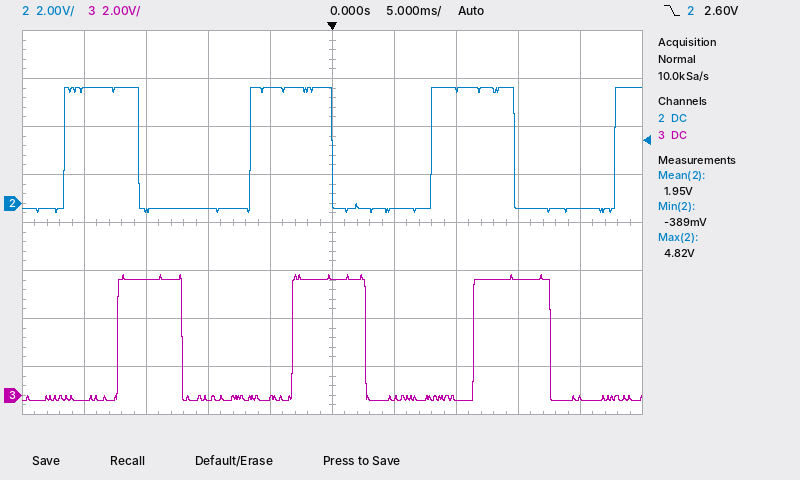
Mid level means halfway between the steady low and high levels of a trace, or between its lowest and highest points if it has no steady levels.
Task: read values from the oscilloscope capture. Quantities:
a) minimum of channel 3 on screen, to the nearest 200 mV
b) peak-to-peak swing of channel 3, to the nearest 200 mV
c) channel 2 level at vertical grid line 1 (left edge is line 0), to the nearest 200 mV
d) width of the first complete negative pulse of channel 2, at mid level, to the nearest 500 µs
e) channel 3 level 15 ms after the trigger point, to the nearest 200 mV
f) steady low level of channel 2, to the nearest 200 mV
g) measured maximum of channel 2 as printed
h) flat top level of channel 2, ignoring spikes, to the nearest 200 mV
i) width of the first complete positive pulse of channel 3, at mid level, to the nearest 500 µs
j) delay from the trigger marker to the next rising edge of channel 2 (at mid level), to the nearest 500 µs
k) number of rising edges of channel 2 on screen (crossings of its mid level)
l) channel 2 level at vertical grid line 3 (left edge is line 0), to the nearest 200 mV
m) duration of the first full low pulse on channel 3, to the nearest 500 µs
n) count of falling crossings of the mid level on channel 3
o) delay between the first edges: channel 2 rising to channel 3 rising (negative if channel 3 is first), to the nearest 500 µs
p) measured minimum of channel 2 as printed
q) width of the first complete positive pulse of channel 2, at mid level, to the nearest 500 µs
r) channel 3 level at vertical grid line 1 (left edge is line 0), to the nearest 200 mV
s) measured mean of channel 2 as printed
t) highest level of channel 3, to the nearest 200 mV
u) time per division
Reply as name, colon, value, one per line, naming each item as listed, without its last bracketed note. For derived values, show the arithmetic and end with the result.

minimum of channel 3 on screen, to the nearest 200 mV: -200 mV
peak-to-peak swing of channel 3, to the nearest 200 mV: 5.0 V − (-200 mV) = 5.2 V
channel 2 level at vertical grid line 1 (left edge is line 0), to the nearest 200 mV: 4.8 V
width of the first complete negative pulse of channel 2, at mid level, to the nearest 500 µs: 9.0 ms
channel 3 level 15 ms after the trigger point, to the nearest 200 mV: 4.8 V
steady low level of channel 2, to the nearest 200 mV: -200 mV
measured maximum of channel 2 as printed: 4.82 V
flat top level of channel 2, ignoring spikes, to the nearest 200 mV: 4.8 V
width of the first complete positive pulse of channel 3, at mid level, to the nearest 500 µs: 5.0 ms
delay from the trigger marker to the next rising edge of channel 2 (at mid level), to the nearest 500 µs: 8.0 ms
number of rising edges of channel 2 on screen: 4
channel 2 level at vertical grid line 3 (left edge is line 0), to the nearest 200 mV: -200 mV
duration of the first full low pulse on channel 3, to the nearest 500 µs: 9.0 ms
count of falling crossings of the mid level on channel 3: 3
delay between the first edges: channel 2 rising to channel 3 rising (negative if channel 3 is first), to the nearest 500 µs: +4.5 ms
measured minimum of channel 2 as printed: -389 mV
width of the first complete positive pulse of channel 2, at mid level, to the nearest 500 µs: 6.0 ms
channel 3 level at vertical grid line 1 (left edge is line 0), to the nearest 200 mV: -200 mV
measured mean of channel 2 as printed: 1.95 V
highest level of channel 3, to the nearest 200 mV: 5.0 V
time per division: 5 ms
